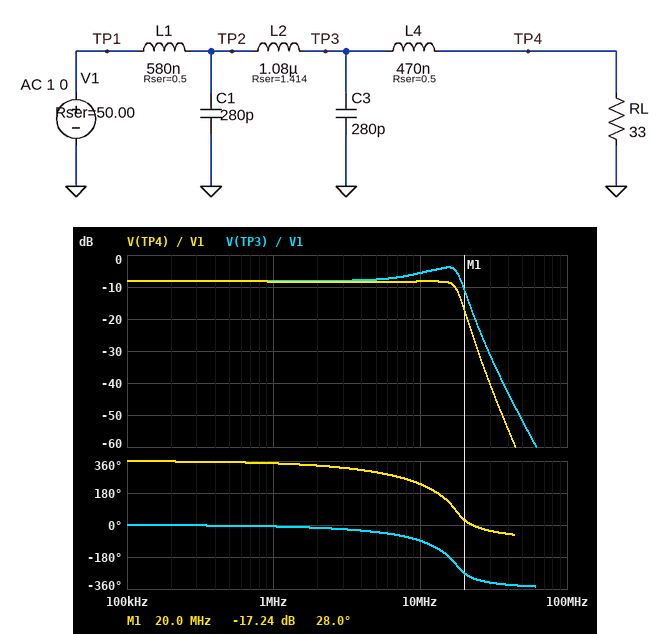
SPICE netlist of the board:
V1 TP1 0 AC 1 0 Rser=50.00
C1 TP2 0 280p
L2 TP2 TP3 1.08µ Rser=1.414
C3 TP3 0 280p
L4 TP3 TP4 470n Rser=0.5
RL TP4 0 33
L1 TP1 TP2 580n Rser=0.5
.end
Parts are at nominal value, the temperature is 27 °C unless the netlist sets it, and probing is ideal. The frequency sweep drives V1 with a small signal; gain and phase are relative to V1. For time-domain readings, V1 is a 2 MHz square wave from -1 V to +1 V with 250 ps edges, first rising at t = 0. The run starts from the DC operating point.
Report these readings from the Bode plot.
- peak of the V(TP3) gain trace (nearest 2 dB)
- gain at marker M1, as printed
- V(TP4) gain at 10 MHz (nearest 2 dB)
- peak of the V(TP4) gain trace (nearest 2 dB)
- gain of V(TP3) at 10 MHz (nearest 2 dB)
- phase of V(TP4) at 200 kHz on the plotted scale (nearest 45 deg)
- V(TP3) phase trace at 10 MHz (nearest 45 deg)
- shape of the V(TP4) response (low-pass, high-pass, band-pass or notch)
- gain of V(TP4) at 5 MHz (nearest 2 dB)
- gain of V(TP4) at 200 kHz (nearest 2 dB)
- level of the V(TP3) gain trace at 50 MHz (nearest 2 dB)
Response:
-4 dB
-17.24 dB
-8 dB
-8 dB
-6 dB
360 deg
-90 deg
low-pass
-8 dB
-8 dB
-52 dB
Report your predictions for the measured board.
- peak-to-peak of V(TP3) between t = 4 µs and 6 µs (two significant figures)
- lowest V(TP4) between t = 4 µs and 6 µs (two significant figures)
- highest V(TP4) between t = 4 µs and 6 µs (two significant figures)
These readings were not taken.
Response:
1.3 V
-500 mV
500 mV
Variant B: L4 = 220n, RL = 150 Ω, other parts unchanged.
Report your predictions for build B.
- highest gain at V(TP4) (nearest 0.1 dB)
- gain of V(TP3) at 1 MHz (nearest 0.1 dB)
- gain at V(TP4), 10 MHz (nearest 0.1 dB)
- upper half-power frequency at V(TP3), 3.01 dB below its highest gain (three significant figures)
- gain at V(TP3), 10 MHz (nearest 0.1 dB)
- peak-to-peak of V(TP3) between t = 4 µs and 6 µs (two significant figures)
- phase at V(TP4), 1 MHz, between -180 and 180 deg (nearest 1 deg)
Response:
-2.1 dB
-2.5 dB
-2.8 dB
15.9 MHz
-2.7 dB
2.0 V
-11 deg
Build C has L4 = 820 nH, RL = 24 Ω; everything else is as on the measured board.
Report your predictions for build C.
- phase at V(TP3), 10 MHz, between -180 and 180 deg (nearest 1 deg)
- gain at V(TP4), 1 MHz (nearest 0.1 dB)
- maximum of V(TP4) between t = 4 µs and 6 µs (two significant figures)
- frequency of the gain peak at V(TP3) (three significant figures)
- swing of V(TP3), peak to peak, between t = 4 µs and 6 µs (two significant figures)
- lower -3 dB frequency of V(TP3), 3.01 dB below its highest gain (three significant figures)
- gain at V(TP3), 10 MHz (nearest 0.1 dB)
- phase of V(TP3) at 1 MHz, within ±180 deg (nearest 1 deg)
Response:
-82 deg
-10.1 dB
390 mV
15.7 MHz
1.7 V
10.8 MHz
-2.6 dB
-3 deg
